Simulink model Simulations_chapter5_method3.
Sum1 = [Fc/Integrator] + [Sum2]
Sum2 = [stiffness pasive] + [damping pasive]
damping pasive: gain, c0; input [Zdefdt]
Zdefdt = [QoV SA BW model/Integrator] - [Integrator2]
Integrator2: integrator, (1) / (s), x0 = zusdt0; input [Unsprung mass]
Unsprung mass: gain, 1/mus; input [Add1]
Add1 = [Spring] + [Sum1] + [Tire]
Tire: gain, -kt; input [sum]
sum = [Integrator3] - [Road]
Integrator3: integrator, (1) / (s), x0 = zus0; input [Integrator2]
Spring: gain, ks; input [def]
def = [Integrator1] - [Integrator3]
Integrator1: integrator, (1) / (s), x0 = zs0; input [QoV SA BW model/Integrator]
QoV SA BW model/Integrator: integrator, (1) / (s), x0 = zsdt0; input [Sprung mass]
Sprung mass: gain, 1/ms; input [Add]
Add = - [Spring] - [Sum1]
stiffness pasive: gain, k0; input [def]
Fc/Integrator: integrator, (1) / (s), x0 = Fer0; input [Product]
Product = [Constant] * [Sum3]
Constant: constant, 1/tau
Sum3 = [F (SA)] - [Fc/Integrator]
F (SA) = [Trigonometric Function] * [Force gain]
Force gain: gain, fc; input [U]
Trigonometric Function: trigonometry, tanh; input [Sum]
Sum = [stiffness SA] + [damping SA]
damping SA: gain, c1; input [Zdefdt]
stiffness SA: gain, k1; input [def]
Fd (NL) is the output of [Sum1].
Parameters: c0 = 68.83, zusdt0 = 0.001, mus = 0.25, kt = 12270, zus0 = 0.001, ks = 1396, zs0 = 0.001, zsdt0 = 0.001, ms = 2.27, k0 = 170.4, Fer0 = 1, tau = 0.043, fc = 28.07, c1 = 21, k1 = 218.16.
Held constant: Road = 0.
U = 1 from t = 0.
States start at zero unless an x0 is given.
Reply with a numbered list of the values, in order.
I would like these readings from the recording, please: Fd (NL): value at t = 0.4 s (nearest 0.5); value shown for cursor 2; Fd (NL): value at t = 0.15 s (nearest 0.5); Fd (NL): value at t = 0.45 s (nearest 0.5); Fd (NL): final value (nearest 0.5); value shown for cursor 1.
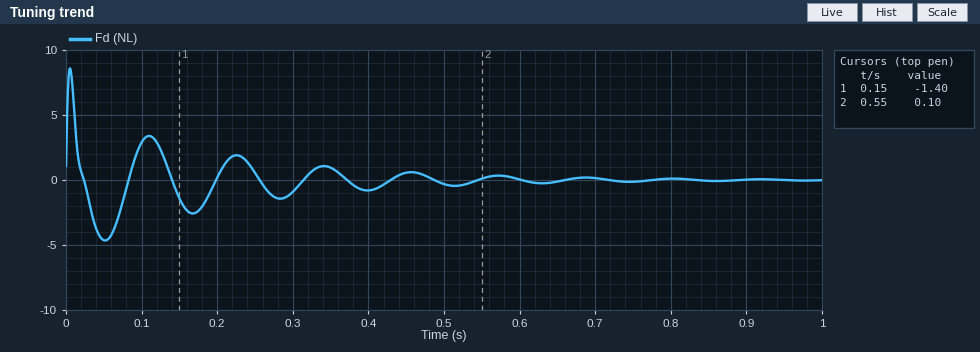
1. -1.0
2. 0.10
3. -1.5
4. 0.5
5. 0.0
6. -1.40
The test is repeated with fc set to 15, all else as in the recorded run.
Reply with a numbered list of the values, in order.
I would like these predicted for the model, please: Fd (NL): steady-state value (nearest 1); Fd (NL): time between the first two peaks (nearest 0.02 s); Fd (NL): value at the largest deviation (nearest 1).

1. 0
2. 0.12 s
3. 8
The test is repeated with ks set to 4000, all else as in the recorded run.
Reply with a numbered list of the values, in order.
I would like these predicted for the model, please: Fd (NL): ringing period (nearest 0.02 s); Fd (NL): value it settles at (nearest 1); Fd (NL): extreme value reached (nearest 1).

1. 0.10 s
2. 0
3. 8
